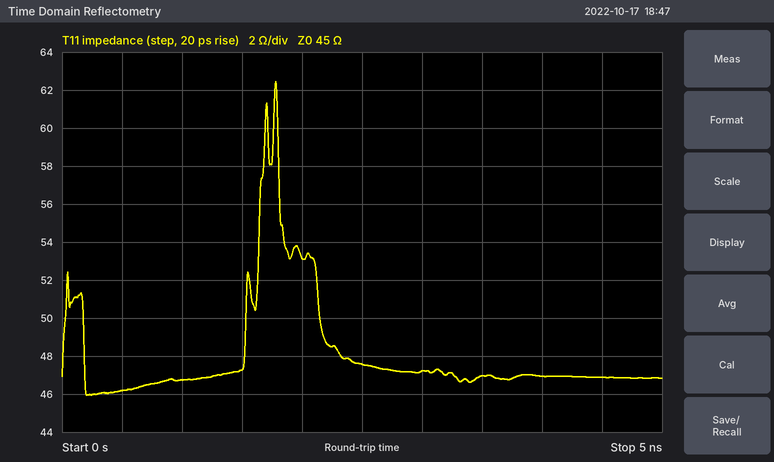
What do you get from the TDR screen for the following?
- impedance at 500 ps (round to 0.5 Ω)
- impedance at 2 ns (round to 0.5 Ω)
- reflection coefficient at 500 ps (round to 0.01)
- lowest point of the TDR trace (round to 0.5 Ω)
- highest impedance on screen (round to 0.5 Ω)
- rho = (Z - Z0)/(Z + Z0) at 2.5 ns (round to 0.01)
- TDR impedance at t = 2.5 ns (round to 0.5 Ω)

46.0 Ω
53.0 Ω
+0.01
46.0 Ω
62.5 Ω
+0.03
47.5 Ω
